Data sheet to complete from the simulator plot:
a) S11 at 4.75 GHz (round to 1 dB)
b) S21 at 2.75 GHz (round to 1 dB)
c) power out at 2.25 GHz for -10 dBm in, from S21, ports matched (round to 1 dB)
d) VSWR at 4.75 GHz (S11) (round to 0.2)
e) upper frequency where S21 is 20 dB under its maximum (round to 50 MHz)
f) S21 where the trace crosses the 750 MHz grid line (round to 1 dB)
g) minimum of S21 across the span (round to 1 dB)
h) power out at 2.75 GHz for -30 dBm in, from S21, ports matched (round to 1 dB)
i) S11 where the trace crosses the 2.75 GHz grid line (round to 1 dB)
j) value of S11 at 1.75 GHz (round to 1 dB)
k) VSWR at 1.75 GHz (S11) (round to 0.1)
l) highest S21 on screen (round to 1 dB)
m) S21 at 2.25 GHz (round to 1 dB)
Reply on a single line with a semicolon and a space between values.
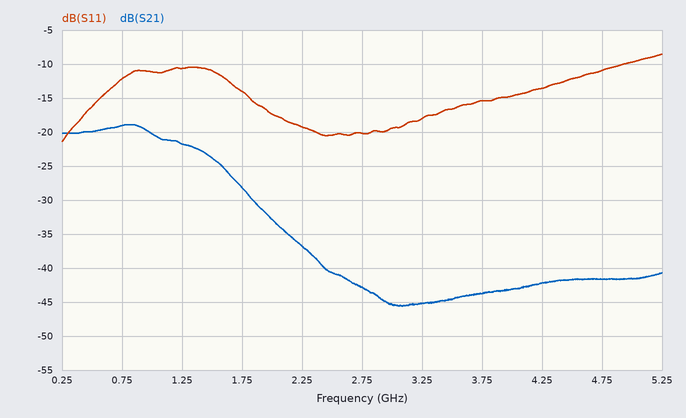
-11 dB; -43 dB; -47 dBm; 1.8; 2.40 GHz; -19 dB; -46 dB; -73 dBm; -20 dB; -14 dB; 1.5; -19 dB; -37 dB
